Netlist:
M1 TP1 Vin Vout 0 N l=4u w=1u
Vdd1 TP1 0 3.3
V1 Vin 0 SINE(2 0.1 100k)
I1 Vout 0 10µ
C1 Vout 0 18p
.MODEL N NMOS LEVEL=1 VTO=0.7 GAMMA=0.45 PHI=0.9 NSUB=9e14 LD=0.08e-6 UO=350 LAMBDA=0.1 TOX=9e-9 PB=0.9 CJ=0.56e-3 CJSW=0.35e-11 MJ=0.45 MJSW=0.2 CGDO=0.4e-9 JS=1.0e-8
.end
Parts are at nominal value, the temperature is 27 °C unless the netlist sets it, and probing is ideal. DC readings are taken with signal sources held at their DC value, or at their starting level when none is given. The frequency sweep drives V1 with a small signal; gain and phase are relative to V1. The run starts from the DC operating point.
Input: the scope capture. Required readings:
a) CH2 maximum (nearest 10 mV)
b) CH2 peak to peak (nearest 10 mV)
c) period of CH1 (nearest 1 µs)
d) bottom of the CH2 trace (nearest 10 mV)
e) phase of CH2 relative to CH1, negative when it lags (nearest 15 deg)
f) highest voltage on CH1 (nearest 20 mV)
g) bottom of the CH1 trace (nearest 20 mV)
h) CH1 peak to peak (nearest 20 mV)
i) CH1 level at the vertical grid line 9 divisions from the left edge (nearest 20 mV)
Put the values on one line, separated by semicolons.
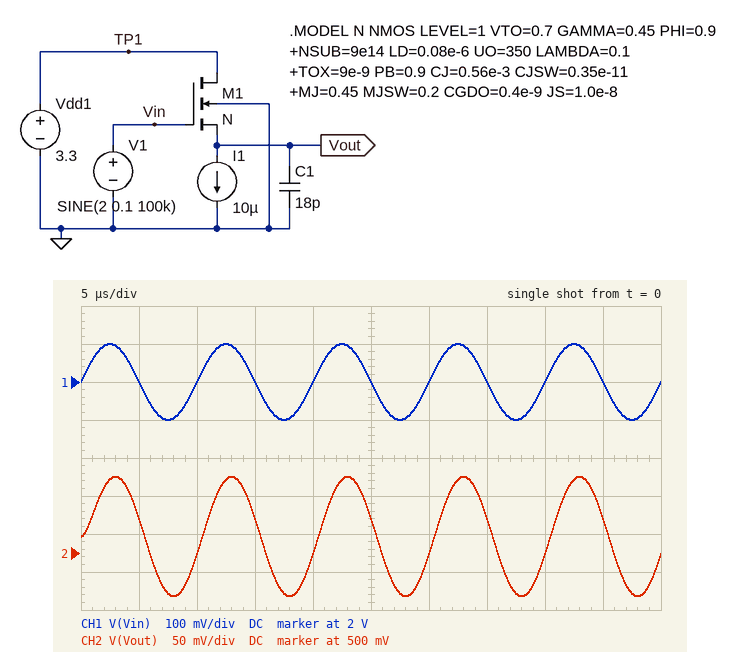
600 mV; 160 mV; 10 µs; 440 mV; -15 deg; 2.10 V; 1.90 V; 200 mV; 2.00 V
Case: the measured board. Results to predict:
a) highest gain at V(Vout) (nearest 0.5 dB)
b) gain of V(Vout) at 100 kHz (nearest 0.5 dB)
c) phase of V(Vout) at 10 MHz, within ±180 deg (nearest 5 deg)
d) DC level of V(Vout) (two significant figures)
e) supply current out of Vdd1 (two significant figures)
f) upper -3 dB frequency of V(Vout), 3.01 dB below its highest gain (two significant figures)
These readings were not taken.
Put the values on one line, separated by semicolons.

-1.5 dB; -2.0 dB; -85 deg; 520 mV; 10 µA; 320 kHz
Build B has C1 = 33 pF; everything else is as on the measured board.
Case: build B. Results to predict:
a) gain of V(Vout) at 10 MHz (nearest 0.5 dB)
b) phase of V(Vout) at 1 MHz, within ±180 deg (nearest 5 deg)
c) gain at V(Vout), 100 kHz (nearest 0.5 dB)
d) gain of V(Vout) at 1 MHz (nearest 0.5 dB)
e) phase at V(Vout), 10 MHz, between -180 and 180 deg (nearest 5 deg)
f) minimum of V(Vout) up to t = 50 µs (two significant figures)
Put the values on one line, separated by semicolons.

-37.0 dB; -80 deg; -3.0 dB; -17.0 dB; -90 deg; 450 mV
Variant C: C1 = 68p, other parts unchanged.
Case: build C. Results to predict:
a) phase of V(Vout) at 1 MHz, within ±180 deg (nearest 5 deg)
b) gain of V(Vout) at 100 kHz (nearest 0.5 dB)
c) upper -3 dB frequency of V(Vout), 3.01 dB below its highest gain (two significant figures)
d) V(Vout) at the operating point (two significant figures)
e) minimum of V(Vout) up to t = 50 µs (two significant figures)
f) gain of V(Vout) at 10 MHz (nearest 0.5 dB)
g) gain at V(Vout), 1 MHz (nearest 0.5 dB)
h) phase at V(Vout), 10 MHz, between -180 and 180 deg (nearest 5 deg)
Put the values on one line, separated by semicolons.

-85 deg; -5.5 dB; 85 kHz; 520 mV; 470 mV; -43.0 dB; -23.0 dB; -90 deg
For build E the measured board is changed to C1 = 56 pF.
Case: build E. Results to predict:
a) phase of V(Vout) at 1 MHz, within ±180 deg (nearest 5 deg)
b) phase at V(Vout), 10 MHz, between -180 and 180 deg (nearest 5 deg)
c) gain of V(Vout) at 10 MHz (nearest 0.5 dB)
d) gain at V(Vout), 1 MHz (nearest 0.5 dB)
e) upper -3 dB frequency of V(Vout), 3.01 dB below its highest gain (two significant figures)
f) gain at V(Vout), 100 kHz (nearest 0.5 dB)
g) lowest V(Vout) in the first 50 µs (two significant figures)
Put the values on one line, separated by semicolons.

-85 deg; -90 deg; -41.5 dB; -21.5 dB; 100 kHz; -4.5 dB; 460 mV
